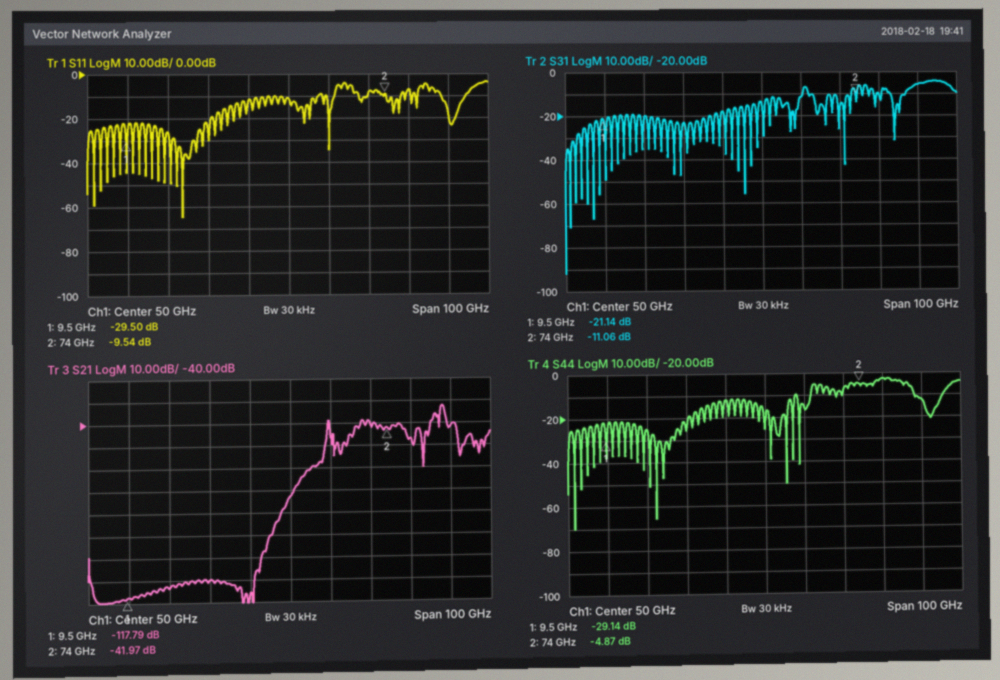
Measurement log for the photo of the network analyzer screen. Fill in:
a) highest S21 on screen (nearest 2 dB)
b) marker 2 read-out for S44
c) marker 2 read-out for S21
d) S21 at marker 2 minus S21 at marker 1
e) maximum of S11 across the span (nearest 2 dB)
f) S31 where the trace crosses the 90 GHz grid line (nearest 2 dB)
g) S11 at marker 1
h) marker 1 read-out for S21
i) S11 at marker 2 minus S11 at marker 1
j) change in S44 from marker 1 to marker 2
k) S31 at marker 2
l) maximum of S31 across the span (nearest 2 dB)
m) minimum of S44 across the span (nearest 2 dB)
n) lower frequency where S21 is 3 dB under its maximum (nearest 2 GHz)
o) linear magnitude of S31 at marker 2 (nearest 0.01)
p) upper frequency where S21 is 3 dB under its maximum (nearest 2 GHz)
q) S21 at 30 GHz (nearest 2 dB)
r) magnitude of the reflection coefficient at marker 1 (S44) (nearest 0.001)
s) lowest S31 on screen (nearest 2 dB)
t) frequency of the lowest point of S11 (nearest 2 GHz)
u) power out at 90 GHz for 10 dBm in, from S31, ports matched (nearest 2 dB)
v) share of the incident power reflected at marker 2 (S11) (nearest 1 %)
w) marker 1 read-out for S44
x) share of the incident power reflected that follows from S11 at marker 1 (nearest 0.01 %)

-32 dB
-4.87 dB
-41.97 dB
75.82 dB
-4 dB
-6 dB
-29.50 dB
-117.79 dB
19.96 dB
24.27 dB
-11.06 dB
-4 dB
-70 dB
88 GHz
0.28
88 GHz
-110 dB
0.035
-92 dB
24 GHz
4 dBm
11 %
-29.14 dB
0.11 %
